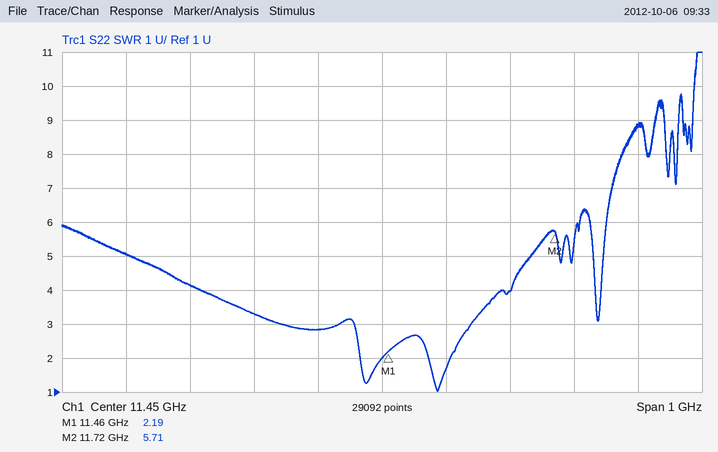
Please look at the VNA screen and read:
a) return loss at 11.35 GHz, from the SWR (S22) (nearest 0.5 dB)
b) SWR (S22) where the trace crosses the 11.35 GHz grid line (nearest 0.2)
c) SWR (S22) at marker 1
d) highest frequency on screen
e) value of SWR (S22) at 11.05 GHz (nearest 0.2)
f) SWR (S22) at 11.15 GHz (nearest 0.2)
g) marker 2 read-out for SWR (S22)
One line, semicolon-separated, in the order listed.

6.5 dB; 2.8; 2.19; 11.95 GHz; 5.0; 4.2; 5.71
